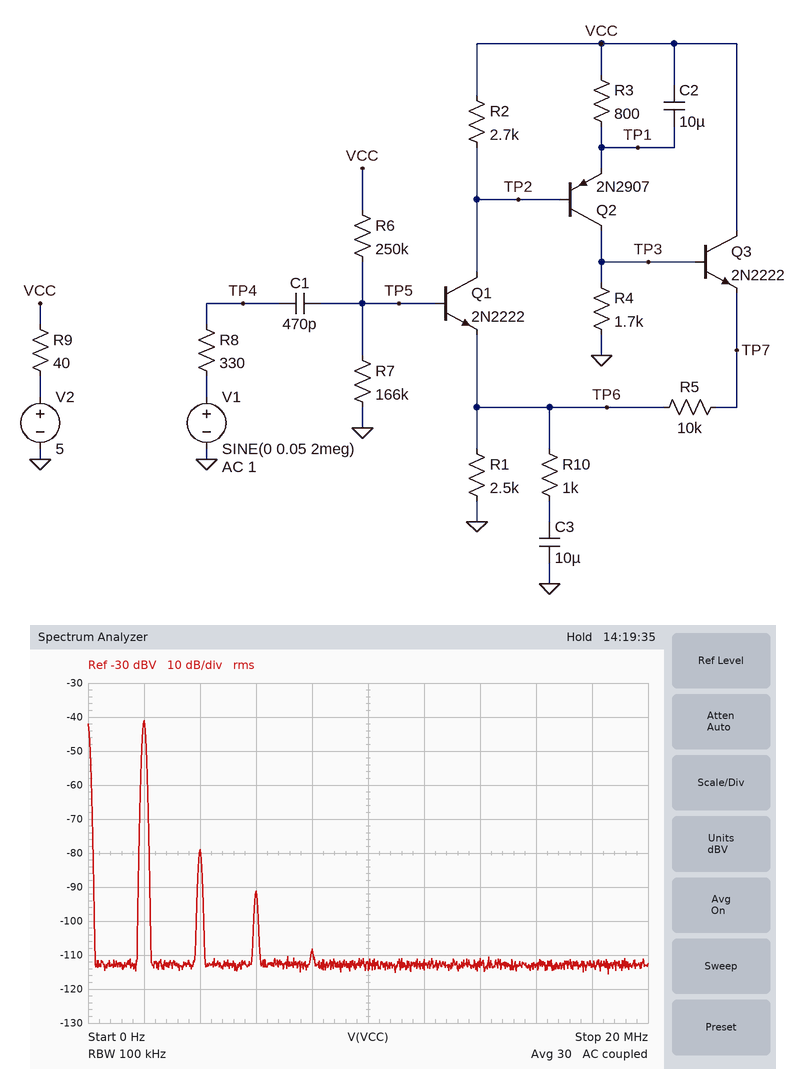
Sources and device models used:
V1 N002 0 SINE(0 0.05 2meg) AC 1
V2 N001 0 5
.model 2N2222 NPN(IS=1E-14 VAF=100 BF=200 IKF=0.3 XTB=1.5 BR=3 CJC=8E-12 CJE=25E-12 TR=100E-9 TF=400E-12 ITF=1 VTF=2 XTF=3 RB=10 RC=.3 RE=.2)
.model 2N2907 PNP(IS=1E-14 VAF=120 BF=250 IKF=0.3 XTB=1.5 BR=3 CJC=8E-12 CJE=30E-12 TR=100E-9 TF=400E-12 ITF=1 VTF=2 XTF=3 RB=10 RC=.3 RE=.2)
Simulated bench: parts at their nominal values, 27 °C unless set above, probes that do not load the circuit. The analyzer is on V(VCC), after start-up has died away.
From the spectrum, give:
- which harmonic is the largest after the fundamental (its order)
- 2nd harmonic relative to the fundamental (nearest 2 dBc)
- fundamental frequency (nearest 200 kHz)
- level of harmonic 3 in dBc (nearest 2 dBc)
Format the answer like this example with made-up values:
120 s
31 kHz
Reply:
2
-38 dBc
2.0 MHz
-50 dBc
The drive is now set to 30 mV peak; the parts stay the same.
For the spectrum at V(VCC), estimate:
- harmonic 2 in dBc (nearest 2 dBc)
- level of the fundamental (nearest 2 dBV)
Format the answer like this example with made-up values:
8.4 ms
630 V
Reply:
-42 dBc
-46 dBV
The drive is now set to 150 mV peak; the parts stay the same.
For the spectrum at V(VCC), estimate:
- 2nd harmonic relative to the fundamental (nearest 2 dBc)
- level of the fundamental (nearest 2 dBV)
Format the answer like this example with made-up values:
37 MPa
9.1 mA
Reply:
-26 dBc
-32 dBV
